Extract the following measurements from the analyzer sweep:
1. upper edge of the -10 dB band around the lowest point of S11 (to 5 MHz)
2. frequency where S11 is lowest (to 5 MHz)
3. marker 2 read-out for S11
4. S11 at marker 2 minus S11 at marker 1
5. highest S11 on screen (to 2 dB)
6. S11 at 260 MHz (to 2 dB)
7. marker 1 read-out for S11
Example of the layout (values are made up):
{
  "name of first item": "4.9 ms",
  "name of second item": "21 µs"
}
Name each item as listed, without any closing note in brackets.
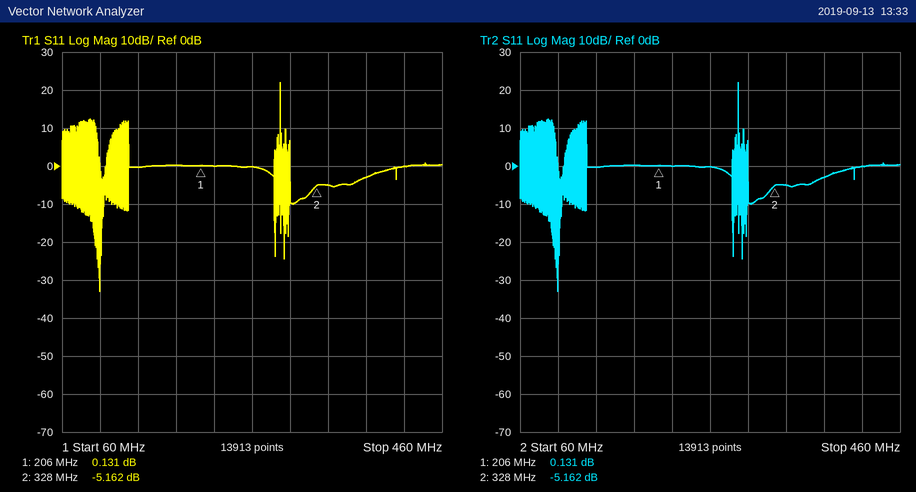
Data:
{
  "upper edge of the -10 dB band around the lowest point of S11": "100 MHz",
  "frequency where S11 is lowest": "100 MHz",
  "marker 2 read-out for S11": "-5.162 dB",
  "S11 at marker 2 minus S11 at marker 1": "-5.293 dB",
  "highest S11 on screen": "22 dB",
  "S11 at 260 MHz": "0 dB",
  "marker 1 read-out for S11": "0.131 dB"
}
